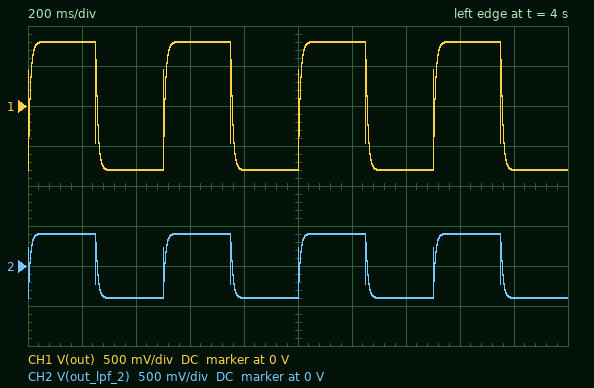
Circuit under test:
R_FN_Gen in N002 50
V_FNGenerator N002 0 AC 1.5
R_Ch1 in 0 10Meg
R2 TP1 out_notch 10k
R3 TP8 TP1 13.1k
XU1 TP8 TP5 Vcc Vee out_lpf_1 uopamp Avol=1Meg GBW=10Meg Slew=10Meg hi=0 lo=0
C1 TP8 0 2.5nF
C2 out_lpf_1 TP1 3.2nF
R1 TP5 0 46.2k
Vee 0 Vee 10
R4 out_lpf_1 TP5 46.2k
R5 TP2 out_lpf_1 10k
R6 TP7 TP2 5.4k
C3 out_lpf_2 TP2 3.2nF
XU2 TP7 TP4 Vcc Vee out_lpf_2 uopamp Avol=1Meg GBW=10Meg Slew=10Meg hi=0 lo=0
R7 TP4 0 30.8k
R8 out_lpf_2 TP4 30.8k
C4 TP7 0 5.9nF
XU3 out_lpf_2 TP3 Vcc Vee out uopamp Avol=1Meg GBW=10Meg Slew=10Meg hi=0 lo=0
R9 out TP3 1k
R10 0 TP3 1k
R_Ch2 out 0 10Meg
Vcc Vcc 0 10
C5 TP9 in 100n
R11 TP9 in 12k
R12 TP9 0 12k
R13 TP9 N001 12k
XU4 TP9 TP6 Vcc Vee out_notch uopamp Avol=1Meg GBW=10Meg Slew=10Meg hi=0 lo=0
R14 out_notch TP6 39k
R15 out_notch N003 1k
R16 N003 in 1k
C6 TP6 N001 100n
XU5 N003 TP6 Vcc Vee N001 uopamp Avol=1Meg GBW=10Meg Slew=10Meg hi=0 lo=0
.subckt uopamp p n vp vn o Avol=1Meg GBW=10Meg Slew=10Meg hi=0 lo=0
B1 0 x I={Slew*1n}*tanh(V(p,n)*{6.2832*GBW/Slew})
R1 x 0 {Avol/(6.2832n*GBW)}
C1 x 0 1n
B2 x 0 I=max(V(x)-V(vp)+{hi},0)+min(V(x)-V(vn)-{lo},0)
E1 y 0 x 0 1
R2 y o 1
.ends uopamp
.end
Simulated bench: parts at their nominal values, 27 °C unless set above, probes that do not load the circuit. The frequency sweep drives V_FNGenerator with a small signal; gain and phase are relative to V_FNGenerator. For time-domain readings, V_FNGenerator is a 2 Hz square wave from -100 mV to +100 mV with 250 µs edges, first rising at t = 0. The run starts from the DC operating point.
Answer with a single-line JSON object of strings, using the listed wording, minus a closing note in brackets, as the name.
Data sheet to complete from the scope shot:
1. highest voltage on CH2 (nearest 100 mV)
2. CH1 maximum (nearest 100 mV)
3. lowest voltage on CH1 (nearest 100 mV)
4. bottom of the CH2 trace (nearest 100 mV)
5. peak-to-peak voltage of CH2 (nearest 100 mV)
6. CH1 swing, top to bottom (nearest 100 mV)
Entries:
{"highest voltage on CH2": "400 mV", "CH1 maximum": "800 mV", "lowest voltage on CH1": "-800 mV", "bottom of the CH2 trace": "-400 mV", "peak-to-peak voltage of CH2": "800 mV", "CH1 swing, top to bottom": "1.6 V"}
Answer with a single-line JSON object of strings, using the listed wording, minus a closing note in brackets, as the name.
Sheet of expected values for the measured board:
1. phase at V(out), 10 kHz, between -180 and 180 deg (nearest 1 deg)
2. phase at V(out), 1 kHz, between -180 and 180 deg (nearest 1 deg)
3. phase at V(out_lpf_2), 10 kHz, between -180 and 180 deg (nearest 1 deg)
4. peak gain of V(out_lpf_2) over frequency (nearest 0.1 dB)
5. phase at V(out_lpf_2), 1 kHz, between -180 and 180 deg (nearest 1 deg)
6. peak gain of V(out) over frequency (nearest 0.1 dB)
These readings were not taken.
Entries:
{"phase at V(out), 10 kHz, between -180 and 180 deg": "79 deg", "phase at V(out), 1 kHz, between -180 and 180 deg": "-15 deg", "phase at V(out_lpf_2), 10 kHz, between -180 and 180 deg": "79 deg", "peak gain of V(out_lpf_2) over frequency": "12.0 dB", "phase at V(out_lpf_2), 1 kHz, between -180 and 180 deg": "-15 deg", "peak gain of V(out) over frequency": "18.1 dB"}
